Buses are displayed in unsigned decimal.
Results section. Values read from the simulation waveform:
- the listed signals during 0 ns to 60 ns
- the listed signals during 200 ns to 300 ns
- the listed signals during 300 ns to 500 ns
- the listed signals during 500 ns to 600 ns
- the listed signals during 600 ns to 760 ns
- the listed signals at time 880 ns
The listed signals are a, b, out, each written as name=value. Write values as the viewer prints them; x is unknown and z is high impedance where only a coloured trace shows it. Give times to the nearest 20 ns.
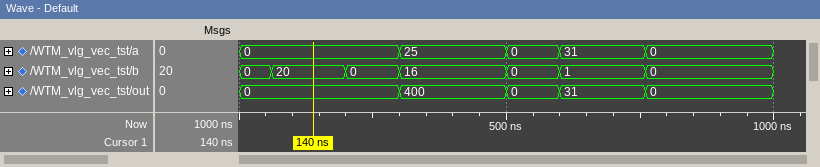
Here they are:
a=0, b=0, out=0
a=0, b=0, out=0
a=25, b=16, out=400
a=0, b=0, out=0
a=31, b=1, out=31
a=0, b=0, out=0
